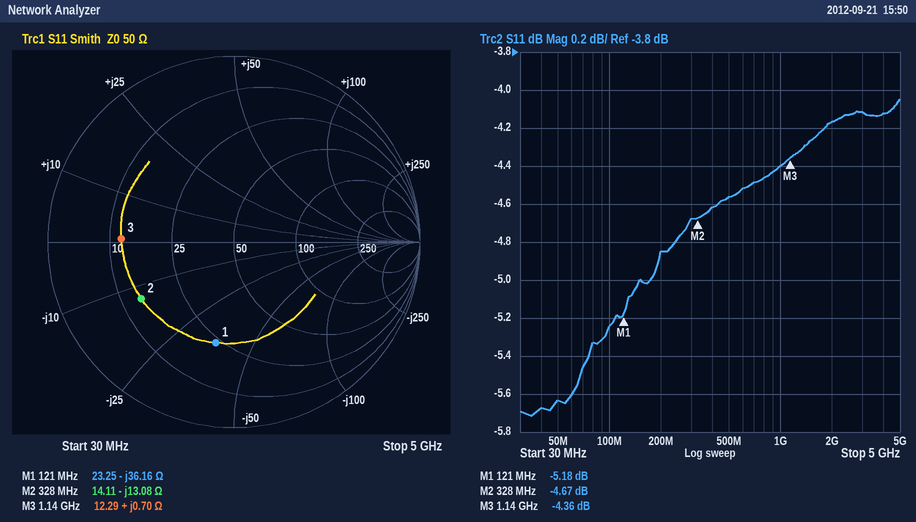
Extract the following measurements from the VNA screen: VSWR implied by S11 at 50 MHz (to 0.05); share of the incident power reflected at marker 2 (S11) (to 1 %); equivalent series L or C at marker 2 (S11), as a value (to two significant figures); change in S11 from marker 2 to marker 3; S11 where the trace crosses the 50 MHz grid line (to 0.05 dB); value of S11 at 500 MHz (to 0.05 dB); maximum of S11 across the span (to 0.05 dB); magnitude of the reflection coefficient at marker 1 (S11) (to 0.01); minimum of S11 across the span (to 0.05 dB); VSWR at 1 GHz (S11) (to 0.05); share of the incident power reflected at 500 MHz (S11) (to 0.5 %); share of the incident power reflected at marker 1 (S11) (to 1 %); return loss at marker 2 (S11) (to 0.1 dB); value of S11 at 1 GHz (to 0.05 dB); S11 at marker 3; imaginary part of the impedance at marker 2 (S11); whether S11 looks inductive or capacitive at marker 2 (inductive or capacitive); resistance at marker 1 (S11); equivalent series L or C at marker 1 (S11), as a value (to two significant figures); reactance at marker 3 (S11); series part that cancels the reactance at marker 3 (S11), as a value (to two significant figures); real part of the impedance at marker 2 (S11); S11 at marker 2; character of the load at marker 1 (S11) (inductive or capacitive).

3.20
34 %
37 pF
0.31 dB
-5.65 dB
-4.55 dB
-4.05 dB
0.55
-5.70 dB
4.05
35.0 %
30 %
4.7 dB
-4.40 dB
-4.36 dB
-13.08 Ω
capacitive
23.25 Ω
36 pF
+0.70 Ω
200 pF
14.11 Ω
-4.67 dB
capacitive
